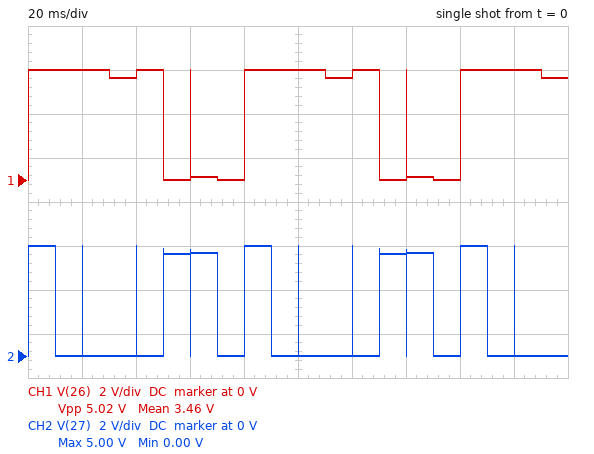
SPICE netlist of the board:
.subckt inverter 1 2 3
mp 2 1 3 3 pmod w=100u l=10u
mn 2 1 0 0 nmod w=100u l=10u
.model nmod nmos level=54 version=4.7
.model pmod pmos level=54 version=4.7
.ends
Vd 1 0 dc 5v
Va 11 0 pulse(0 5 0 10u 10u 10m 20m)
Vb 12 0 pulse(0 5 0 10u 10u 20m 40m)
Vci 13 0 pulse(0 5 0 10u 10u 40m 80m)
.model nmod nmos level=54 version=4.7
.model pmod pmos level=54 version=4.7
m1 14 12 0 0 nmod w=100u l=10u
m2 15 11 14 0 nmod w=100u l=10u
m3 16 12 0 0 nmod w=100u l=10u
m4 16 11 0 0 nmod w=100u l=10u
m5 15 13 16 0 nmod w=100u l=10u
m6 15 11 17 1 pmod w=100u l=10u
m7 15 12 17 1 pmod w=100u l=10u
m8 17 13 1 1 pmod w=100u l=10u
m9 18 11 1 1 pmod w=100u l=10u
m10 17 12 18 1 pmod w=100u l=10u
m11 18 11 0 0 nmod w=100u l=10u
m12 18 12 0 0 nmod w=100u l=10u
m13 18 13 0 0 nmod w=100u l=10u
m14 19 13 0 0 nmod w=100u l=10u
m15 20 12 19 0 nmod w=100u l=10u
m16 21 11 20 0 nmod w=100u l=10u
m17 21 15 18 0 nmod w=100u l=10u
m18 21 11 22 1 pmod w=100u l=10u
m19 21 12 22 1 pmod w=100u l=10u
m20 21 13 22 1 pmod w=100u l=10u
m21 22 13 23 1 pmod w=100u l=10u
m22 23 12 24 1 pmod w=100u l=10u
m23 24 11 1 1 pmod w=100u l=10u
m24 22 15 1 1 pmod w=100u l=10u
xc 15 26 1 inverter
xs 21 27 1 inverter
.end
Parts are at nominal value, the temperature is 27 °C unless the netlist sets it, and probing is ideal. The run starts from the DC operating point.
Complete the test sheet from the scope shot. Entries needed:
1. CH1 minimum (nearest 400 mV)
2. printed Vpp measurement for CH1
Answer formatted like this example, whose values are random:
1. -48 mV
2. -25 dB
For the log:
1. 0 V
2. 5.02 V
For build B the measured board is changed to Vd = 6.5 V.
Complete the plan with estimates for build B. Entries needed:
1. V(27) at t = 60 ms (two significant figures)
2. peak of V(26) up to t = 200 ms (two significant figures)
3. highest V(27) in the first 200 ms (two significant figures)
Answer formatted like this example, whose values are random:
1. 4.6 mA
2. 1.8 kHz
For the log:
1. 5.1 V
2. 6.5 V
3. 6.3 V
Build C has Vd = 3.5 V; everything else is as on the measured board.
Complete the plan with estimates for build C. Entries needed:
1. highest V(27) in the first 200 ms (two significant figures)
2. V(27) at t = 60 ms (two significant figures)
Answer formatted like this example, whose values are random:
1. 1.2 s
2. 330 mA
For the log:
1. 3.5 V
2. 3.4 V
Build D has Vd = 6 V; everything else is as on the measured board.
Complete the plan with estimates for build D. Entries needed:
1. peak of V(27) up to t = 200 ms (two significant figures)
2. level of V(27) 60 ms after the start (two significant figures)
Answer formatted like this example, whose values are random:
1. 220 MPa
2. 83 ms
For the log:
1. 6.0 V
2. 5.1 V
